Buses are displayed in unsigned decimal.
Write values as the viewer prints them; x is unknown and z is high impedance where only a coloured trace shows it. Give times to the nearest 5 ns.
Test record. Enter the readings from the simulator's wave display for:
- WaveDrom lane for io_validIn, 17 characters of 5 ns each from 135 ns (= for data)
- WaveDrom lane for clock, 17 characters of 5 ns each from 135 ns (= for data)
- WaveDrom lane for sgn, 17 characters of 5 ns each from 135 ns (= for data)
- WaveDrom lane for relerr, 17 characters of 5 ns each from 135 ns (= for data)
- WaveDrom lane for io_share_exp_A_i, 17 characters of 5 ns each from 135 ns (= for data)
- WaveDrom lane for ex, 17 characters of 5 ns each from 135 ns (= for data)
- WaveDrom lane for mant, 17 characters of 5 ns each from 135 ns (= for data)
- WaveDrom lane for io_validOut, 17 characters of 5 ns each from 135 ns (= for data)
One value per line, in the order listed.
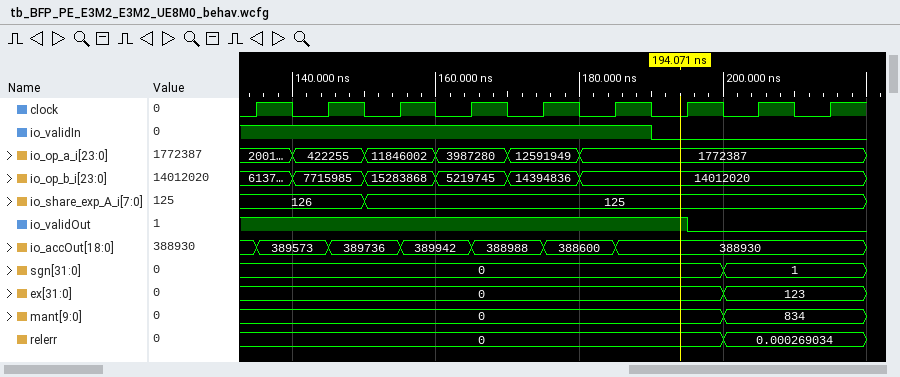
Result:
{name: 'io_validIn', wave: '1..........0.....'}
{name: 'clock', wave: '10101010101010101'}
{name: 'sgn', wave: '=............=...', data: '0 1'}
{name: 'relerr', wave: '=............=...', data: '0 0.000269034'}
{name: 'io_share_exp_A_i', wave: '=..=.............', data: '126 125'}
{name: 'ex', wave: '=............=...', data: '0 123'}
{name: 'mant', wave: '=............=...', data: '0 834'}
{name: 'io_validOut', wave: '1...........0....'}
